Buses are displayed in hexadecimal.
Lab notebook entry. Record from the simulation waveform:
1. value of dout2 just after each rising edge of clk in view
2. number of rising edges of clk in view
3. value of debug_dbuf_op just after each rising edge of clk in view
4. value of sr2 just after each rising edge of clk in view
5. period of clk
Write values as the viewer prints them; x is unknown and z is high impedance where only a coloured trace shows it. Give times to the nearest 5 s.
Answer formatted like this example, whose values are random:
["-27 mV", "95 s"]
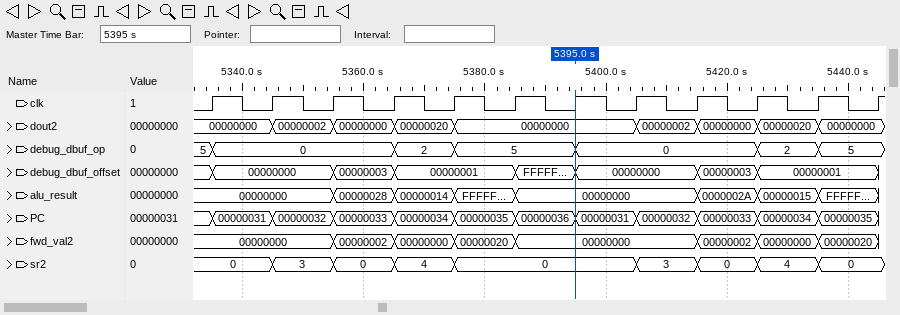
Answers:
["00000000, 00000002, 00000000, 00000020, 00000000, 00000000, 00000000, 00000002, 00000000, 00000020, 00000000, 00000000", "12", "0, 0, 0, 2, 5, 5, 0, 0, 0, 2, 5, 5", "0, 3, 0, 4, 0, 0, 0, 3, 0, 4, 0, 0", "10 s"]
